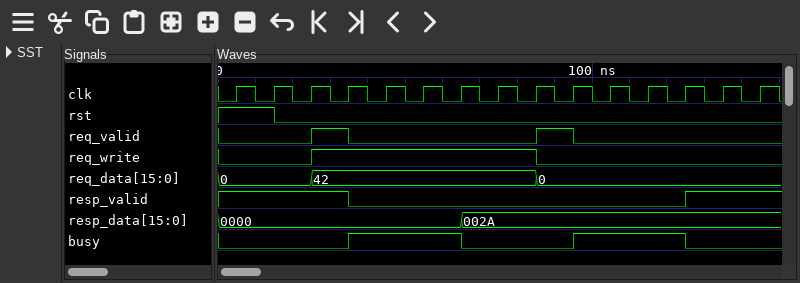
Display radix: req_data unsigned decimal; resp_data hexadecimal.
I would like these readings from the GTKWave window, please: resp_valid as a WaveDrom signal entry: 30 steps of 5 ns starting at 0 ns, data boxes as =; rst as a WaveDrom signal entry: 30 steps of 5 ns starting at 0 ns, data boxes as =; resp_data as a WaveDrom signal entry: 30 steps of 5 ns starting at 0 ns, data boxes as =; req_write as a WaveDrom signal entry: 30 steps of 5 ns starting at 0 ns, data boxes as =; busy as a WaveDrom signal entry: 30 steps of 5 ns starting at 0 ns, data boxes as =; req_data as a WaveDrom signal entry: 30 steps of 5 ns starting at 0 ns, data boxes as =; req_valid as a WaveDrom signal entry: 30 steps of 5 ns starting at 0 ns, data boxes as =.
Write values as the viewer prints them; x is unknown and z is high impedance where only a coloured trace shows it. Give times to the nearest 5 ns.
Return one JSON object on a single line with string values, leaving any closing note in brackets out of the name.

{"resp_valid as a WaveDrom signal entry: 30 steps of 5 ns starting at 0 ns, data boxes as =": "{name: 'resp_valid', wave: '1......0.................1....'}", "rst as a WaveDrom signal entry: 30 steps of 5 ns starting at 0 ns, data boxes as =": "{name: 'rst', wave: '1..0..........................'}", "resp_data as a WaveDrom signal entry: 30 steps of 5 ns starting at 0 ns, data boxes as =": "{name: 'resp_data', wave: '=............=................', data: '0000 002A'}", "req_write as a WaveDrom signal entry: 30 steps of 5 ns starting at 0 ns, data boxes as =": "{name: 'req_write', wave: '0....1...........0............'}", "busy as a WaveDrom signal entry: 30 steps of 5 ns starting at 0 ns, data boxes as =": "{name: 'busy', wave: '0......1.....0.....1.....0....'}", "req_data as a WaveDrom signal entry: 30 steps of 5 ns starting at 0 ns, data boxes as =": "{name: 'req_data', wave: '=....=...........=............', data: '0 42 0'}", "req_valid as a WaveDrom signal entry: 30 steps of 5 ns starting at 0 ns, data boxes as =": "{name: 'req_valid', wave: '0....1.0.........1.0..........'}"}
